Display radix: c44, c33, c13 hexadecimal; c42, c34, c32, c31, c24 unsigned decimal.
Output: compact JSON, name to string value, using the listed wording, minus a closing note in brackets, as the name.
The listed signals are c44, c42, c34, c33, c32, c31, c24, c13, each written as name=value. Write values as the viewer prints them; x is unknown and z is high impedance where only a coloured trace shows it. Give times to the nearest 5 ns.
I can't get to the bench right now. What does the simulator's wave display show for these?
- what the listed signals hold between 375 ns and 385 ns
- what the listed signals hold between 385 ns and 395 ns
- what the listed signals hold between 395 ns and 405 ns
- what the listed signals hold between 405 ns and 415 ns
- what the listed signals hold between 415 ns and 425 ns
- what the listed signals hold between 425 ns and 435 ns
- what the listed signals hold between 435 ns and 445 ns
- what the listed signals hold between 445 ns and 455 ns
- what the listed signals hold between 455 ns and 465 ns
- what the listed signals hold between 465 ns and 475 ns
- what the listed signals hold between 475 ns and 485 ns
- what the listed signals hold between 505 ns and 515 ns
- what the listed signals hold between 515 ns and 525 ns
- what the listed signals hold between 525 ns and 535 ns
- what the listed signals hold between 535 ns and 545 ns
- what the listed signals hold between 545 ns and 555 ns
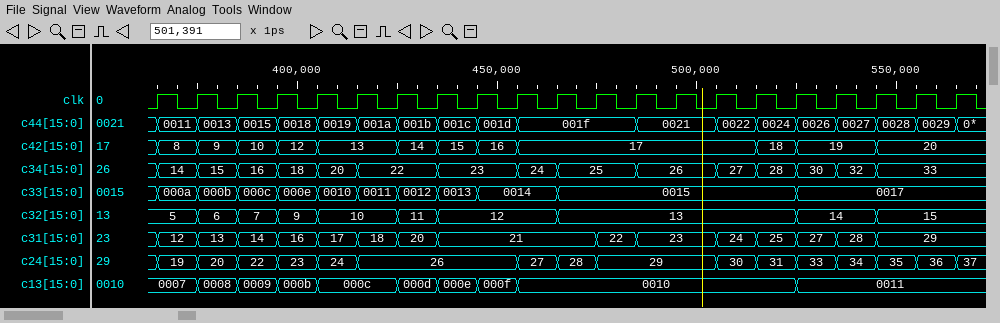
{"what the listed signals hold between 375 ns and 385 ns": "c44=0013, c42=9, c34=15, c33=000b, c32=6, c31=13, c24=20, c13=0008", "what the listed signals hold between 385 ns and 395 ns": "c44=0015, c42=10, c34=16, c33=000c, c32=7, c31=14, c24=22, c13=0009", "what the listed signals hold between 395 ns and 405 ns": "c44=0018, c42=12, c34=18, c33=000e, c32=9, c31=16, c24=23, c13=000b", "what the listed signals hold between 405 ns and 415 ns": "c44=0019, c42=13, c34=20, c33=0010, c32=10, c31=17, c24=24, c13=000c", "what the listed signals hold between 415 ns and 425 ns": "c44=001a, c42=13, c34=22, c33=0011, c32=10, c31=18, c24=26, c13=000c", "what the listed signals hold between 425 ns and 435 ns": "c44=001b, c42=14, c34=22, c33=0012, c32=11, c31=20, c24=26, c13=000d", "what the listed signals hold between 435 ns and 445 ns": "c44=001c, c42=15, c34=23, c33=0013, c32=12, c31=21, c24=26, c13=000e", "what the listed signals hold between 445 ns and 455 ns": "c44=001d, c42=16, c34=23, c33=0014, c32=12, c31=21, c24=26, c13=000f", "what the listed signals hold between 455 ns and 465 ns": "c44=001f, c42=17, c34=24, c33=0014, c32=12, c31=21, c24=27, c13=0010", "what the listed signals hold between 465 ns and 475 ns": "c44=001f, c42=17, c34=25, c33=0015, c32=13, c31=21, c24=28, c13=0010", "what the listed signals hold between 475 ns and 485 ns": "c44=001f, c42=17, c34=25, c33=0015, c32=13, c31=22, c24=29, c13=0010", "what the listed signals hold between 505 ns and 515 ns": "c44=0022, c42=17, c34=27, c33=0015, c32=13, c31=24, c24=30, c13=0010", "what the listed signals hold between 515 ns and 525 ns": "c44=0024, c42=18, c34=28, c33=0015, c32=13, c31=25, c24=31, c13=0010", "what the listed signals hold between 525 ns and 535 ns": "c44=0026, c42=19, c34=30, c33=0017, c32=14, c31=27, c24=33, c13=0011", "what the listed signals hold between 535 ns and 545 ns": "c44=0027, c42=19, c34=32, c33=0017, c32=14, c31=28, c24=34, c13=0011", "what the listed signals hold between 545 ns and 555 ns": "c44=0028, c42=20, c34=33, c33=0017, c32=15, c31=29, c24=35, c13=0011"}
